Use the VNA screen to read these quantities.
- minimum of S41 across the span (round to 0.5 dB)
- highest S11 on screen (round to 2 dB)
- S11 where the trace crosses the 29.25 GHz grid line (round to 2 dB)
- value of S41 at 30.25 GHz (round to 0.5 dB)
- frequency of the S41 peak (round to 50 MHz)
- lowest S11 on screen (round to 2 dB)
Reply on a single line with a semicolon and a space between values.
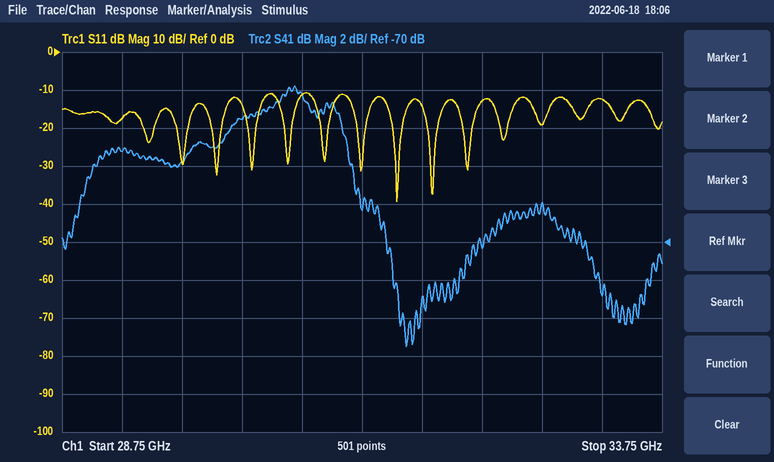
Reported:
-75.5 dB; -10 dB; -18 dB; -63.5 dB; 30.70 GHz; -40 dB
